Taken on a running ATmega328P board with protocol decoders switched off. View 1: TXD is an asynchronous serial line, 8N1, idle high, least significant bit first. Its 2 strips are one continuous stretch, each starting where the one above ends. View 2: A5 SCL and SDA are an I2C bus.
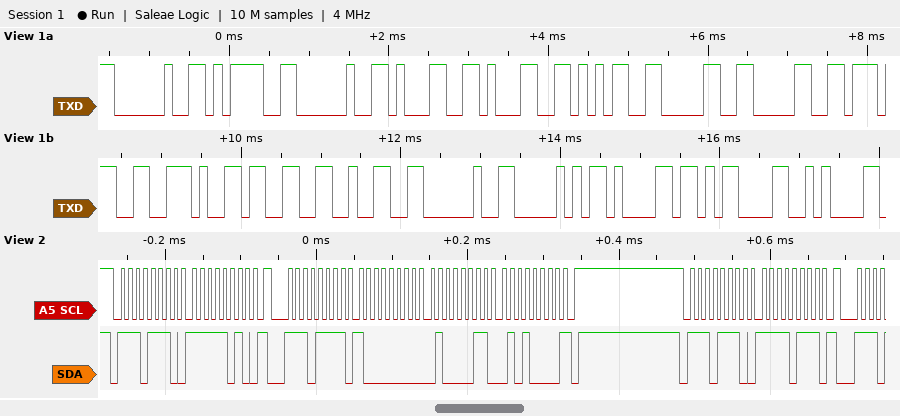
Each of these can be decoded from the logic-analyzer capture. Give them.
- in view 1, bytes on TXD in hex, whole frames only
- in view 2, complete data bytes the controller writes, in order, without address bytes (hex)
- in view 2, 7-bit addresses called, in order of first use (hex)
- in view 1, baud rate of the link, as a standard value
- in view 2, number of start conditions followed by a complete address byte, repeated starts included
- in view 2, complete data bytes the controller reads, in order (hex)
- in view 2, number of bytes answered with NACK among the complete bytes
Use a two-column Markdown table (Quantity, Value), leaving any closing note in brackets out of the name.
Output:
| Quantity | Value |
|---|---|
| in view 1, bytes on TXD in hex, whole frames only | 20 3D 20 31 31 35 30 30 37 2E 33 32 20 50 61 0D 0A |
| in view 2, complete data bytes the controller writes, in order, without address bytes | FA F7 |
| in view 2, 7-bit addresses called, in order of first use | 0x77 |
| in view 1, baud rate of the link, as a standard value | 9600 baud |
| in view 2, number of start conditions followed by a complete address byte, repeated starts included | 3 |
| in view 2, complete data bytes the controller reads, in order | 80 43 50 |
| in view 2, number of bytes answered with NACK among the complete bytes | 1 |
